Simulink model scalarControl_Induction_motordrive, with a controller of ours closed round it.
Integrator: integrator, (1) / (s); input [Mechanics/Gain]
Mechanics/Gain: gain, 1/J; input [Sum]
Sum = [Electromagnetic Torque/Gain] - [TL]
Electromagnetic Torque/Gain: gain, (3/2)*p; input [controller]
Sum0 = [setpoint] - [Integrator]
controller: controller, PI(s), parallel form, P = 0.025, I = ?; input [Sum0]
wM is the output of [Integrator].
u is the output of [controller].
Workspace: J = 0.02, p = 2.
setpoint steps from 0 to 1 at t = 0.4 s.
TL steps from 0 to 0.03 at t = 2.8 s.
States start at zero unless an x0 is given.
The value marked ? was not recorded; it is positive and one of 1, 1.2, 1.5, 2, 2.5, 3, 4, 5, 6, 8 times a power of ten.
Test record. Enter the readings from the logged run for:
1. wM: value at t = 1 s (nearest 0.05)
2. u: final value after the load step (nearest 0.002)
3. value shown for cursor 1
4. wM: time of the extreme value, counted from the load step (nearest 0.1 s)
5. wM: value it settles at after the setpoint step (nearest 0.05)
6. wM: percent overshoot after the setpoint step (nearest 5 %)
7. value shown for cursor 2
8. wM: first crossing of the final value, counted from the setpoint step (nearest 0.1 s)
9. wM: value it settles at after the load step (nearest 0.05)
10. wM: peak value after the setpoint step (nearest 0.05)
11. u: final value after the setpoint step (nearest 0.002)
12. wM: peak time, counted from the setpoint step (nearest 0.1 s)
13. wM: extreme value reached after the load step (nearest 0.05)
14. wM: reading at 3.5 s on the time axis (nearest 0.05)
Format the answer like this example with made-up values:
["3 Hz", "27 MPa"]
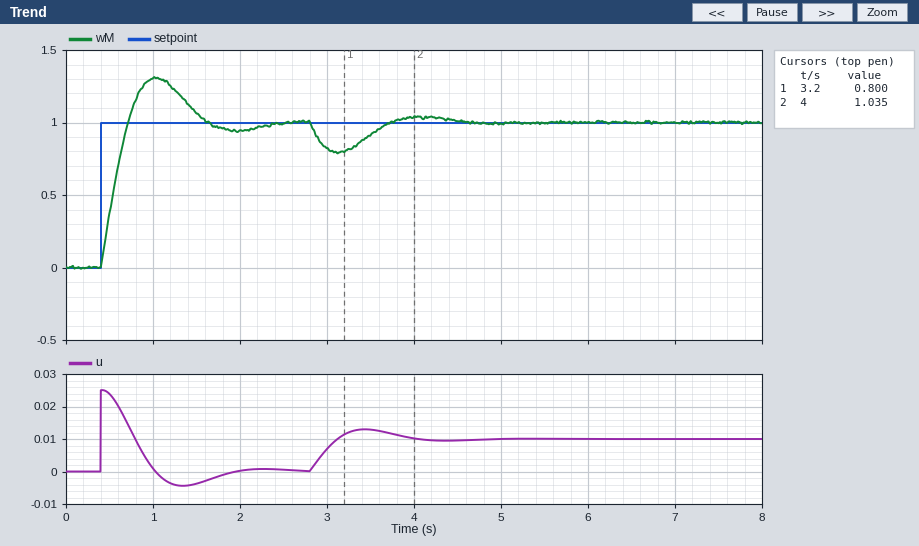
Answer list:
["1.30", "0.010", "0.800", "0.3 s", "1.00", "30 %", "1.035", "0.3 s", "1.00", "1.30", "0.000", "0.6 s", "0.80", "0.90"]
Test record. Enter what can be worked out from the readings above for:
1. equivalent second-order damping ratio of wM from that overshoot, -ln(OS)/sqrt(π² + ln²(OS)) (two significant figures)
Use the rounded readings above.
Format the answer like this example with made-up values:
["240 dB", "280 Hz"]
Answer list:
["0.36"]
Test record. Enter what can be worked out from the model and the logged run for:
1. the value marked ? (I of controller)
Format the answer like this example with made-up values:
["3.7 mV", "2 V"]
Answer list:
["0.1"]
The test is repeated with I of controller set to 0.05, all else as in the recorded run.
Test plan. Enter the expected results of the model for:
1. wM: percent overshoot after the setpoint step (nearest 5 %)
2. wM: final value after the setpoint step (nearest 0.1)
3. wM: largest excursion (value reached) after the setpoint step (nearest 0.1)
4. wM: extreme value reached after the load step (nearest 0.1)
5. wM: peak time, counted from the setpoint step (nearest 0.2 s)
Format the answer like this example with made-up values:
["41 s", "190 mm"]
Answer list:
["20 %", "1.0", "1.2", "0.7", "0.8 s"]
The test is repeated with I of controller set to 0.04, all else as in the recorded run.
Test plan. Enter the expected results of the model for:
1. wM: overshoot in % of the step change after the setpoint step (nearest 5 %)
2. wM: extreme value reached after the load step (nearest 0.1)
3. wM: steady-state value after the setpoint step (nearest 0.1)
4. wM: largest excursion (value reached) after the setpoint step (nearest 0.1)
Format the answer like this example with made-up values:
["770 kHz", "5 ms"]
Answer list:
["20 %", "0.7", "1.0", "1.2"]
